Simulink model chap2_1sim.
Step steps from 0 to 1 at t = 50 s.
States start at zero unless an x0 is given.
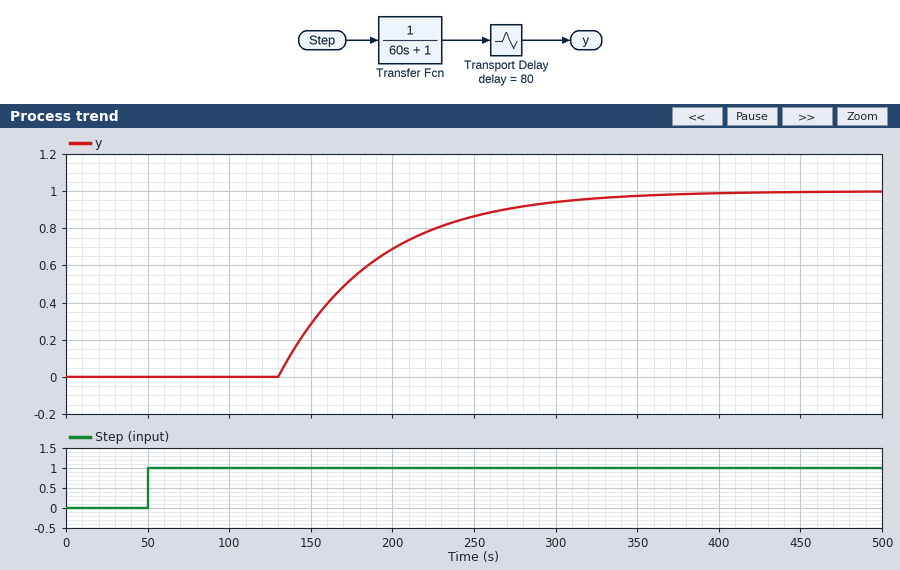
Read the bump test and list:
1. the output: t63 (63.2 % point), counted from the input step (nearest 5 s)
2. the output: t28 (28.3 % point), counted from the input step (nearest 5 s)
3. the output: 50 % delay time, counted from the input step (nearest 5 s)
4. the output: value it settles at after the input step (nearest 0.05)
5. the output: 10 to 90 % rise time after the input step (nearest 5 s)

140 s
100 s
120 s
1.00
130 s
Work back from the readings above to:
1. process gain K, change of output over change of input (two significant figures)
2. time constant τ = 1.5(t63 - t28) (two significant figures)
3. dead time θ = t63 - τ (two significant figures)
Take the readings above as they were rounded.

1.0
60 s
80 s
